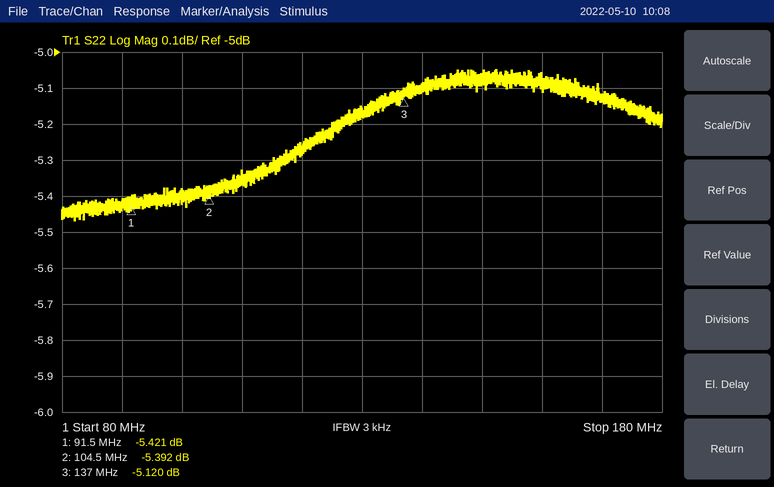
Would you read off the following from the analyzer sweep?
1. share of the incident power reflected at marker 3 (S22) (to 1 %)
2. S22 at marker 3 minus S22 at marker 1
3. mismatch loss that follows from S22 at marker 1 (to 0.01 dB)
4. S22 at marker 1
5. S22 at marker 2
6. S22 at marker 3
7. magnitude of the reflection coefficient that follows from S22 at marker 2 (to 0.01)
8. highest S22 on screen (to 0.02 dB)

31 %
0.301 dB
1.47 dB
-5.421 dB
-5.392 dB
-5.120 dB
0.54
-5.04 dB
